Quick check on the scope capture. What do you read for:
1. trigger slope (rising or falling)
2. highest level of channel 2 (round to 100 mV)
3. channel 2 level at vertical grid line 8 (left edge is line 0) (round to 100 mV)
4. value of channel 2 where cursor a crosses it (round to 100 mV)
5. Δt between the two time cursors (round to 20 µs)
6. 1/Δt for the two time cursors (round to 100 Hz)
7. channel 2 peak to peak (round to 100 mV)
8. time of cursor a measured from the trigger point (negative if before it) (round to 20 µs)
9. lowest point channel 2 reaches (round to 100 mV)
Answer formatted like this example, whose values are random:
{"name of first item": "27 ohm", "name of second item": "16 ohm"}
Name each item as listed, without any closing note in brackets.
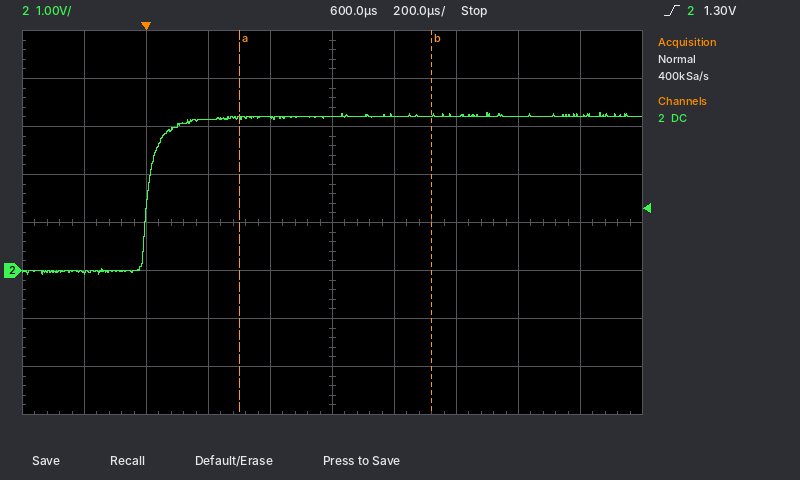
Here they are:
{"trigger slope": "rising", "highest level of channel 2": "3.3 V", "channel 2 level at vertical grid line 8 (left edge is line 0)": "3.2 V", "value of channel 2 where cursor a crosses it": "3.2 V", "Δt between the two time cursors": "620 µs", "1/Δt for the two time cursors": "1.6 kHz", "channel 2 peak to peak": "3.4 V", "time of cursor a measured from the trigger point (negative if before it)": "+300 µs", "lowest point channel 2 reaches": "-100 mV"}
